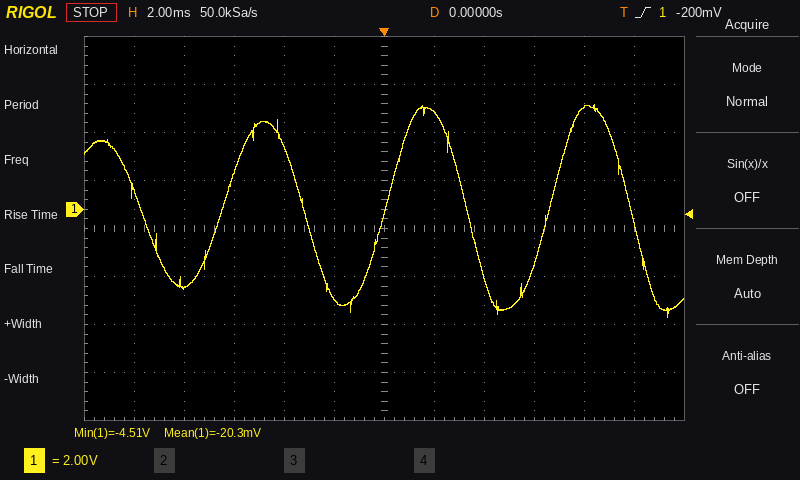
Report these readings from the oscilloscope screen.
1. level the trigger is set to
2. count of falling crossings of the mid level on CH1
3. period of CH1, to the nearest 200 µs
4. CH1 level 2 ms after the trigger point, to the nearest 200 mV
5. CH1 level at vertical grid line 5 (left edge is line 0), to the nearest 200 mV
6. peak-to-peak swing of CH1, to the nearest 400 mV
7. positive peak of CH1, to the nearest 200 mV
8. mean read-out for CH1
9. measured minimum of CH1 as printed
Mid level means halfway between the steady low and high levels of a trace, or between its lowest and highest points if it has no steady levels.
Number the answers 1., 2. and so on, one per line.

1. -200 mV
2. 4
3. 6.6 ms
4. 4.0 V
5. -3.8 V
6. 8.8 V
7. 4.4 V
8. -20.3 mV
9. -4.51 V
